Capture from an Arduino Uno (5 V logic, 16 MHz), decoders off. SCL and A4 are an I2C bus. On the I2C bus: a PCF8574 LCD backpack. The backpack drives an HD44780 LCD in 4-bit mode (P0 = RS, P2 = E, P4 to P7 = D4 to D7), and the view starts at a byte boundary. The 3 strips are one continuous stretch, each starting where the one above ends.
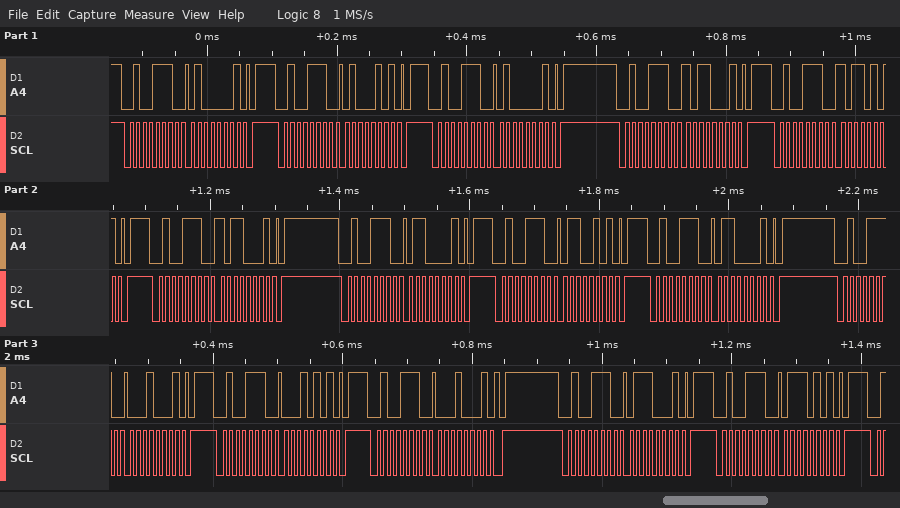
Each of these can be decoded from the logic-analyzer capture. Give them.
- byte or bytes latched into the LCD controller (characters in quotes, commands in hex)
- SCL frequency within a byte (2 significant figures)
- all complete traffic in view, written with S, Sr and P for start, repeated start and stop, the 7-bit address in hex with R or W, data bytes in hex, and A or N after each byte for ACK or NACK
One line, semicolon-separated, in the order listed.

'K' 'a'; 100 kHz; S 27W A 41 A P S 27W A 45 A P S 27W A 41 A P S 27W A B1 A P S 27W A B5 A P S 27W A B1 A P S 27W A 61 A P S 27W A 65 A P S 27W A 61 A P S 27W A 11 A P S 27W A 15 A P S 27W A 11 A P S 27W A 71 A P S 27W A 75 A P
